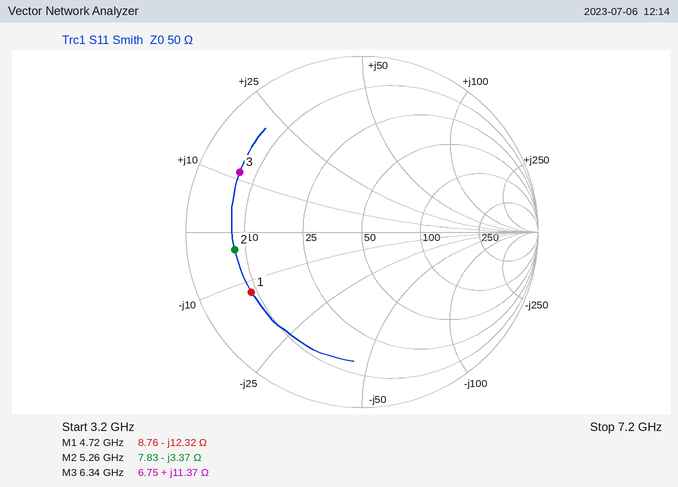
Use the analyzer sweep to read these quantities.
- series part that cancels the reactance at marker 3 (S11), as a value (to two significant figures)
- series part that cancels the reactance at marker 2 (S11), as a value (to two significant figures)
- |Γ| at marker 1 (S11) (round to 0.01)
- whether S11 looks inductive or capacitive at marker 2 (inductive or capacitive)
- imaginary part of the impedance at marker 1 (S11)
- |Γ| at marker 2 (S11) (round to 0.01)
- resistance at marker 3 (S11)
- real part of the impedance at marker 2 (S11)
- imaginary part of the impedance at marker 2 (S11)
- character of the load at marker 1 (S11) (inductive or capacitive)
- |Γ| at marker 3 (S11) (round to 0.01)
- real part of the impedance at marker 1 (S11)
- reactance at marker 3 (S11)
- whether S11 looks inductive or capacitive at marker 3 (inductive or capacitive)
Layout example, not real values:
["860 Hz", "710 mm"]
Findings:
["2.2 pF", "100 pH", "0.72", "capacitive", "-12.32 Ω", "0.73", "6.75 Ω", "7.83 Ω", "-3.37 Ω", "capacitive", "0.77", "8.76 Ω", "+11.37 Ω", "inductive"]
